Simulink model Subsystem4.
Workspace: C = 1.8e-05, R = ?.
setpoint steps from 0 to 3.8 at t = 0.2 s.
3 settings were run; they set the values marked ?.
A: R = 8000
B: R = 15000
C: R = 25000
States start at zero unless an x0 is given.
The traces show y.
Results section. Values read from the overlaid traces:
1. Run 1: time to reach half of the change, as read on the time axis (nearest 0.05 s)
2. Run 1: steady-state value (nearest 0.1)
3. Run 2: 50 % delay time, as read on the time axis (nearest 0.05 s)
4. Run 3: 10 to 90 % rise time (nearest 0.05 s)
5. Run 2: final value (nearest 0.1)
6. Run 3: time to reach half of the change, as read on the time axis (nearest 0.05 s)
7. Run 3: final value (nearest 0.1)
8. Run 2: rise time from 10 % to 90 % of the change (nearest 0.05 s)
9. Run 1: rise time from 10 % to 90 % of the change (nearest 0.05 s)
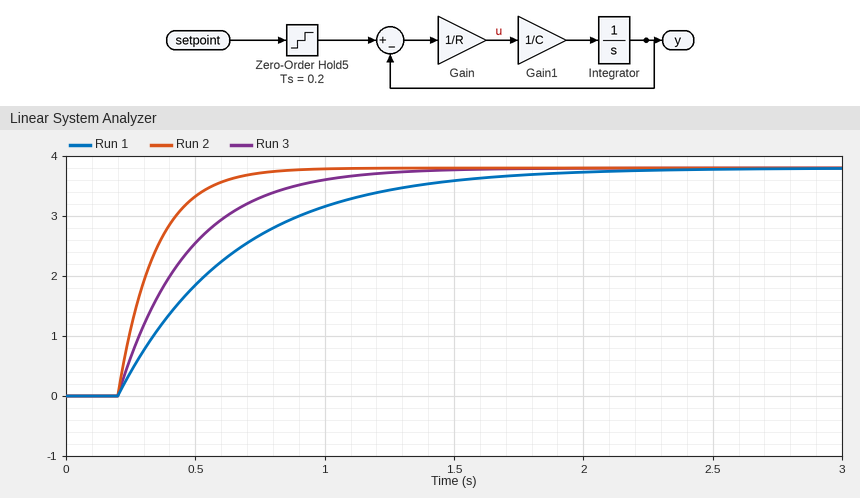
0.50 s
3.8
0.30 s
0.60 s
3.8
0.40 s
3.8
0.30 s
1.00 s
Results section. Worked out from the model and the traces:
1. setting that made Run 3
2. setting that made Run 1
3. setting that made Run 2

B
C
A
